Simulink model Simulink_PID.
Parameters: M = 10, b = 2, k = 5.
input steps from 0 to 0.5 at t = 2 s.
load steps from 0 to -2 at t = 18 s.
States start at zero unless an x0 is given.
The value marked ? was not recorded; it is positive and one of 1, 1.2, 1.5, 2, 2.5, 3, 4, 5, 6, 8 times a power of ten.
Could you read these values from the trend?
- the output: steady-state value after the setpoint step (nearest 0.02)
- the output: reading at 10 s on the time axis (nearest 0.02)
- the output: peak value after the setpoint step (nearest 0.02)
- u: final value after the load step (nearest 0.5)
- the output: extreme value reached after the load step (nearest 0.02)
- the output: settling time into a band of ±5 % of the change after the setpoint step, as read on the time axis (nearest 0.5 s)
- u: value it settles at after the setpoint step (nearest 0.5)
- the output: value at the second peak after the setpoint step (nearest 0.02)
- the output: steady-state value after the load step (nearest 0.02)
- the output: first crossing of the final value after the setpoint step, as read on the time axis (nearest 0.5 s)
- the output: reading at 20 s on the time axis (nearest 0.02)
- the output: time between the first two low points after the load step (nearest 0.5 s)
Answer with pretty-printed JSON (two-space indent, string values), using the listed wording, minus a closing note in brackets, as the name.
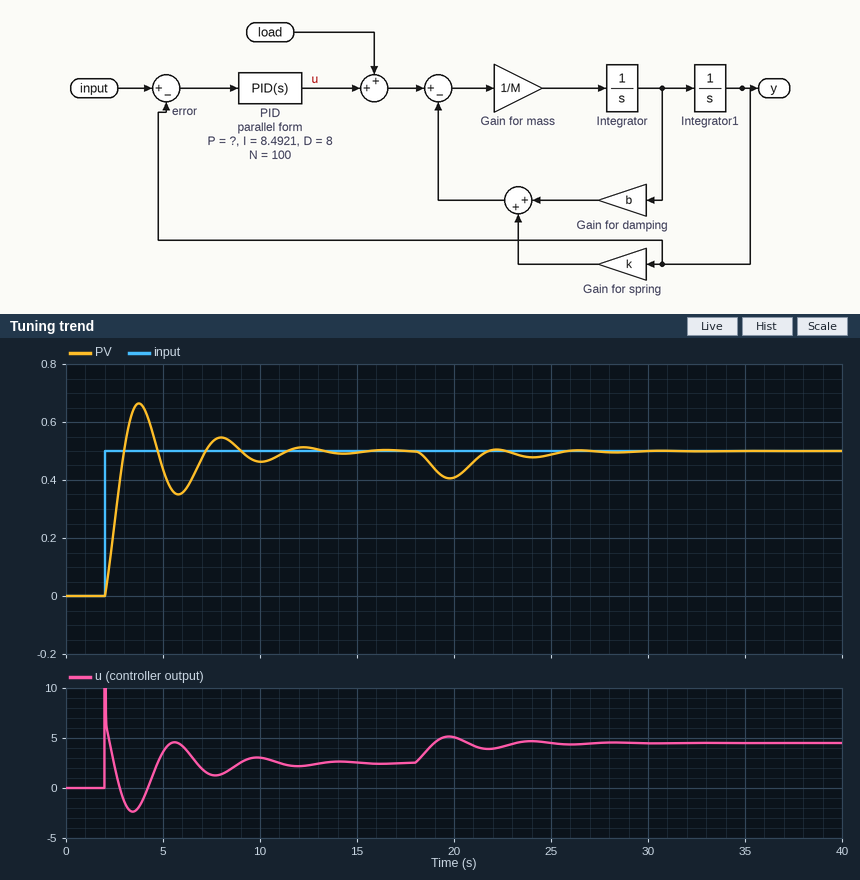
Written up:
{
  "the output: steady-state value after the setpoint step": "0.50",
  "the output: reading at 10 s on the time axis": "0.46",
  "the output: peak value after the setpoint step": "0.66",
  "u: final value after the load step": "4.5",
  "the output: extreme value reached after the load step": "0.40",
  "the output: settling time into a band of ±5 % of the change after the setpoint step, as read on the time axis": "10.5 s",
  "u: value it settles at after the setpoint step": "2.5",
  "the output: value at the second peak after the setpoint step": "0.54",
  "the output: steady-state value after the load step": "0.50",
  "the output: first crossing of the final value after the setpoint step, as read on the time axis": "3.0 s",
  "the output: reading at 20 s on the time axis": "0.40",
  "the output: time between the first two low points after the load step": "4.5 s"
}
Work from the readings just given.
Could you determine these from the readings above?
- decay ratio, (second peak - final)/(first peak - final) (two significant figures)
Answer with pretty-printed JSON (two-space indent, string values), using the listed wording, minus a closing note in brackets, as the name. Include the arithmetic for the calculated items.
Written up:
{
  "decay ratio, (second peak - final)/(first peak - final)": "(0.54 - 0.5) / (0.66 - 0.5) = 0.25"
}
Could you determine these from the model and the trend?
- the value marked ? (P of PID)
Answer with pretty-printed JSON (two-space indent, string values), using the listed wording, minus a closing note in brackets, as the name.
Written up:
{
  "the value marked ?": "20"
}
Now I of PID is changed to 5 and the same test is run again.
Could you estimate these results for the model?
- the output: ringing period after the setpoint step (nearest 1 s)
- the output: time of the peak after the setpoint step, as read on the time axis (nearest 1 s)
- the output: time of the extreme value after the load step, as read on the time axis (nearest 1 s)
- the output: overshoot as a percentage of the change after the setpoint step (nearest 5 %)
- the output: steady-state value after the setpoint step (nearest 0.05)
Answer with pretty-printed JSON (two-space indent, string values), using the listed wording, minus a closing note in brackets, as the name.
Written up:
{
  "the output: ringing period after the setpoint step": "4 s",
  "the output: time of the peak after the setpoint step, as read on the time axis": "4 s",
  "the output: time of the extreme value after the load step, as read on the time axis": "20 s",
  "the output: overshoot as a percentage of the change after the setpoint step": "25 %",
  "the output: steady-state value after the setpoint step": "0.50"
}
